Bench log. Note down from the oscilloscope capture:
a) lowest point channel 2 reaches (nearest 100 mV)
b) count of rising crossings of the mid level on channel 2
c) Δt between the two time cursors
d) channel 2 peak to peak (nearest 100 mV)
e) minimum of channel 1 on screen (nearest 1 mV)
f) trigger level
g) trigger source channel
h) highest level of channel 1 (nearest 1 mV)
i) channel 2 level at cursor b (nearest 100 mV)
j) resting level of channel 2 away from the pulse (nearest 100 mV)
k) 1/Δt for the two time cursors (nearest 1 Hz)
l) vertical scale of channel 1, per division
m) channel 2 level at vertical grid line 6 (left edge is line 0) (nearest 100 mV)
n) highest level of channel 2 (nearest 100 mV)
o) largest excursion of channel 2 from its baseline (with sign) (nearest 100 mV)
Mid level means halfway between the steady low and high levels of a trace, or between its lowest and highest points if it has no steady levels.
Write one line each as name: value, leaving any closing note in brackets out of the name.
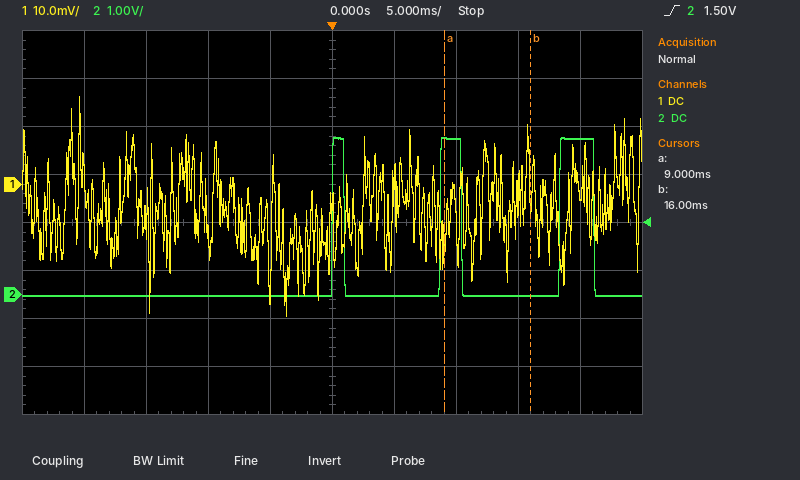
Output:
lowest point channel 2 reaches: 0.0 V
count of rising crossings of the mid level on channel 2: 3
Δt between the two time cursors: 7.0 ms
channel 2 peak to peak: 3.3 V
minimum of channel 1 on screen: -27 mV
trigger level: 1.50 V
trigger source channel: channel 2
highest level of channel 1: 18 mV
channel 2 level at cursor b: 0.0 V
resting level of channel 2 away from the pulse: 0.0 V
1/Δt for the two time cursors: 143 Hz
vertical scale of channel 1, per division: 10 mV
channel 2 level at vertical grid line 6 (left edge is line 0): 0.0 V
highest level of channel 2: 3.3 V
largest excursion of channel 2 from its baseline (with sign): +3.3 V
